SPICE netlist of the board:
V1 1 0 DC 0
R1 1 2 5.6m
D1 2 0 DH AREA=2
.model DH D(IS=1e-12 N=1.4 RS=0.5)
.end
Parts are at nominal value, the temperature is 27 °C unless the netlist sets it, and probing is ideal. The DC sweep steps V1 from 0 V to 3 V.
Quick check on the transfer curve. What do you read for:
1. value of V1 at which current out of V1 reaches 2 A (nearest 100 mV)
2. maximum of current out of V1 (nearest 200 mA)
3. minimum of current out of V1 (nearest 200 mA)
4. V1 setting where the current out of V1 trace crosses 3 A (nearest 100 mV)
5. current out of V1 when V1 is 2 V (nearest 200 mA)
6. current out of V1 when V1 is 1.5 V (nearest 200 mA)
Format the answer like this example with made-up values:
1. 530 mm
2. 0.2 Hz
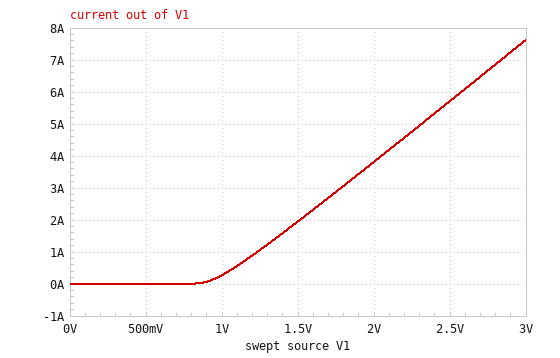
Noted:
1. 1.5 V
2. 7.6 A
3. 0 A
4. 1.8 V
5. 3.8 A
6. 2.0 A
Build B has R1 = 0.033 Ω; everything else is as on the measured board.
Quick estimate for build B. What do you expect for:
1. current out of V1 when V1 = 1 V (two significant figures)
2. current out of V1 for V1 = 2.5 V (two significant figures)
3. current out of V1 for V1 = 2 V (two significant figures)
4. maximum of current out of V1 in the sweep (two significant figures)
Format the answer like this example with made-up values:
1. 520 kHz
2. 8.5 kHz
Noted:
1. 260 mA
2. 5.2 A
3. 3.5 A
4. 6.9 A
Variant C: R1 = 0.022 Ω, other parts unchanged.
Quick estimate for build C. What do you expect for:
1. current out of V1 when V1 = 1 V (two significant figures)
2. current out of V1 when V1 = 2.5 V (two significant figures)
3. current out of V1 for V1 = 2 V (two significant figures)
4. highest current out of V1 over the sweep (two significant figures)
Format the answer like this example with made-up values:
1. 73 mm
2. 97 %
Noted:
1. 270 mA
2. 5.4 A
3. 3.6 A
4. 7.2 A
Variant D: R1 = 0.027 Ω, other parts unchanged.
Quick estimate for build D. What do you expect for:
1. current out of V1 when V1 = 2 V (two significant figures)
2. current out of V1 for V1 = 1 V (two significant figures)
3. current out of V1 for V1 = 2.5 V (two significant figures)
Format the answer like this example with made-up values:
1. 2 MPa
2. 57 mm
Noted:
1. 3.5 A
2. 260 mA
3. 5.3 A
